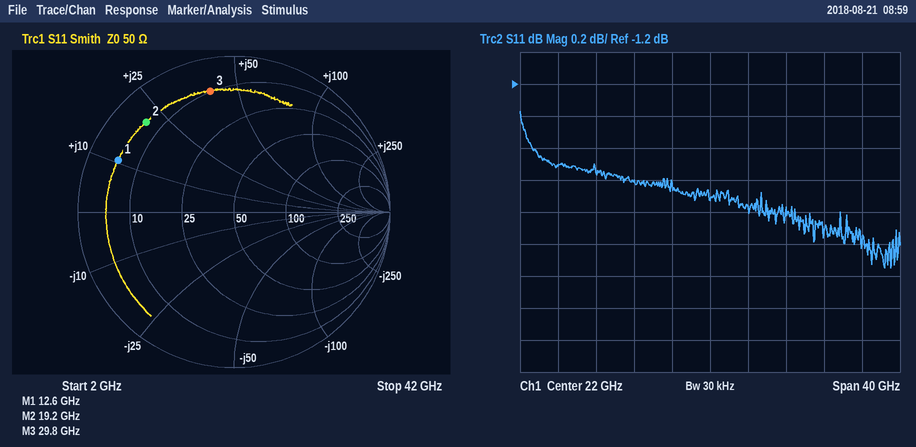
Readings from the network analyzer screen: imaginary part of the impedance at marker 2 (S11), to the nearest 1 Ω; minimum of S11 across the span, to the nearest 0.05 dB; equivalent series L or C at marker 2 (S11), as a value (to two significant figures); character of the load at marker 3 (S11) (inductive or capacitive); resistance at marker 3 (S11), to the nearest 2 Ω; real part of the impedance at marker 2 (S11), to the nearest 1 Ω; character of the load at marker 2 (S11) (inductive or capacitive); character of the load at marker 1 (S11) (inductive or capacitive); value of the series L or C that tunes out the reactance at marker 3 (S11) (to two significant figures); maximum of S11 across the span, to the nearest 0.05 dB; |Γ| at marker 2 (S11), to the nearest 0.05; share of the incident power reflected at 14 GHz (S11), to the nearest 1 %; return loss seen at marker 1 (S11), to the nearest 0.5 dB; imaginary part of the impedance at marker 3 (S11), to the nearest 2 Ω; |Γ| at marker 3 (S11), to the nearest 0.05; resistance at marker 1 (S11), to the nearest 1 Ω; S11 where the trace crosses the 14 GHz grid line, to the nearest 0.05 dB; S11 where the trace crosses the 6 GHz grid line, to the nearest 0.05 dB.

+21 Ω
-2.35 dB
170 pH
inductive
10 Ω
6 Ω
inductive
inductive
130 fF
-1.35 dB
0.80
66 %
2.0 dB
+40 Ω
0.80
5 Ω
-1.80 dB
-1.70 dB
